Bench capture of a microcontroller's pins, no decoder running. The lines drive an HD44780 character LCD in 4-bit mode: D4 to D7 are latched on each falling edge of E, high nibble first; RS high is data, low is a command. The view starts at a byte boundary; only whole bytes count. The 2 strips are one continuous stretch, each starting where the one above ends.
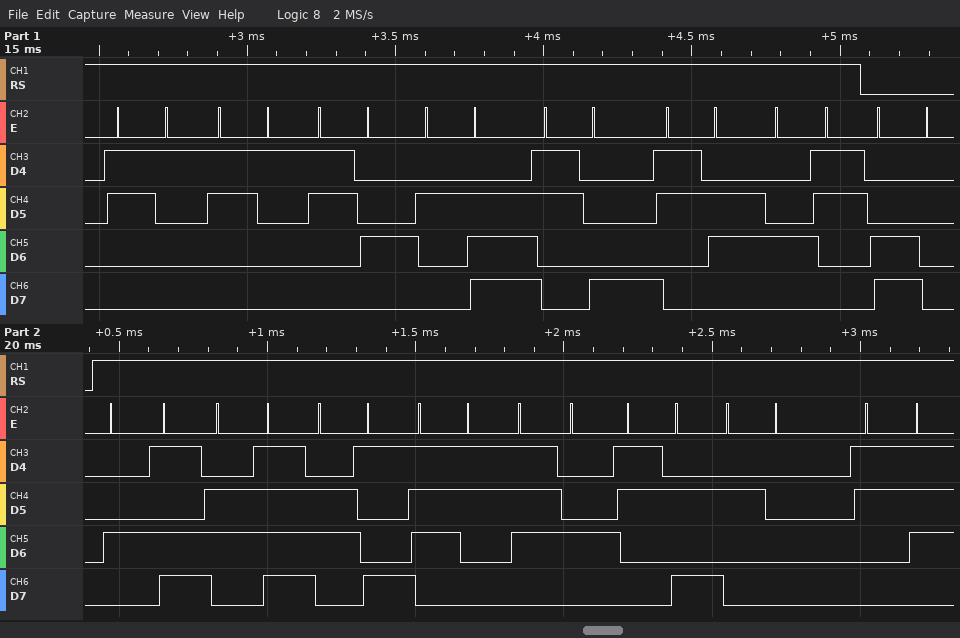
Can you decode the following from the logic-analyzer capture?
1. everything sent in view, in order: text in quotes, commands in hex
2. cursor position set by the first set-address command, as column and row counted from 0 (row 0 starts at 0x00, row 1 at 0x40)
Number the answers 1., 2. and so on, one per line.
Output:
1. "114.86C" 0xC0 "Moist: 7"
2. column 0, row 1
